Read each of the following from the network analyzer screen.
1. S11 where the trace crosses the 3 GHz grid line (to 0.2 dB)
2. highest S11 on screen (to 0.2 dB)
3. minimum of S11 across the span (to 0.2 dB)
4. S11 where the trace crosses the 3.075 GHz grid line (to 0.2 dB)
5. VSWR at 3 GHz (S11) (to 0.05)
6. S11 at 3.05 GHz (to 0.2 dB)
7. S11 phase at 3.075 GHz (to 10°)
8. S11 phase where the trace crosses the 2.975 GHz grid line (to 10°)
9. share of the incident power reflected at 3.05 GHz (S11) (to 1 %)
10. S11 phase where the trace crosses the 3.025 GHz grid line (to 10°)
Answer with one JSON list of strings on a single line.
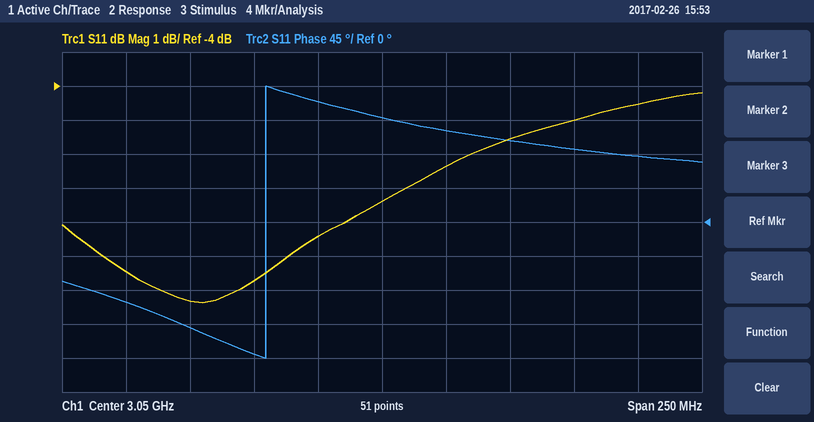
["-9.8 dB", "-4.2 dB", "-10.4 dB", "-6.4 dB", "1.95", "-7.4 dB", "120°", "-140°", "18 %", "160°"]
